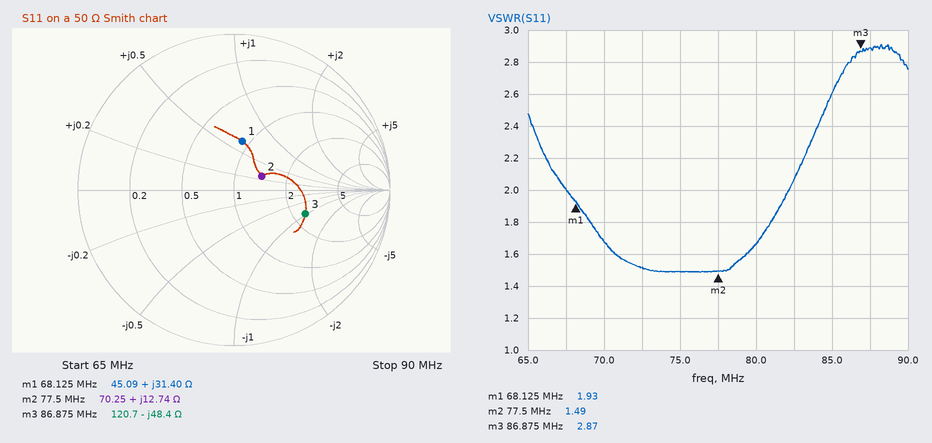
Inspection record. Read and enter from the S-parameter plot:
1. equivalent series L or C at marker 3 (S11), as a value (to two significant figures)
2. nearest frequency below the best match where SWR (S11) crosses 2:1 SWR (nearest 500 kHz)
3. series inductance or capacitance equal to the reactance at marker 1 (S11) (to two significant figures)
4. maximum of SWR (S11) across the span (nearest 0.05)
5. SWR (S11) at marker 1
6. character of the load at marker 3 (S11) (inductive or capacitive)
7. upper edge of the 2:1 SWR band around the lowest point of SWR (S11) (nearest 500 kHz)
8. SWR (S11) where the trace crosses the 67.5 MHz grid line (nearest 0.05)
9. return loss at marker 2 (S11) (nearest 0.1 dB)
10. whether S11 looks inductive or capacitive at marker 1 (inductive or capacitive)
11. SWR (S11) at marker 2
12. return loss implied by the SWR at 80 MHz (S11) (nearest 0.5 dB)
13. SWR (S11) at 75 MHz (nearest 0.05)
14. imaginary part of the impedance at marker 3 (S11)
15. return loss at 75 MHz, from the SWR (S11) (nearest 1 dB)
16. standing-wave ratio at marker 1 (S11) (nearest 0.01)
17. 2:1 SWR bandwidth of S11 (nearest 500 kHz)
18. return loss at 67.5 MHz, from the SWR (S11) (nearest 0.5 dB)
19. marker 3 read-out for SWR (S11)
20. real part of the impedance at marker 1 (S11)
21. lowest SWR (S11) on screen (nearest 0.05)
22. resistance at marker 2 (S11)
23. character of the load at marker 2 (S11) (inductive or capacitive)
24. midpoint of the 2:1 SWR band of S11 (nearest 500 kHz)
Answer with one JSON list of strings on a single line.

["38 pF", "67.5 MHz", "73 nH", "2.90", "1.93", "capacitive", "82.0 MHz", "2.00", "14.1 dB", "inductive", "1.49", "12.0 dB", "1.50", "-48.4 Ω", "14 dB", "1.93", "14.5 MHz", "9.5 dB", "2.87", "45.09 Ω", "1.50", "70.25 Ω", "inductive", "75.0 MHz"]
